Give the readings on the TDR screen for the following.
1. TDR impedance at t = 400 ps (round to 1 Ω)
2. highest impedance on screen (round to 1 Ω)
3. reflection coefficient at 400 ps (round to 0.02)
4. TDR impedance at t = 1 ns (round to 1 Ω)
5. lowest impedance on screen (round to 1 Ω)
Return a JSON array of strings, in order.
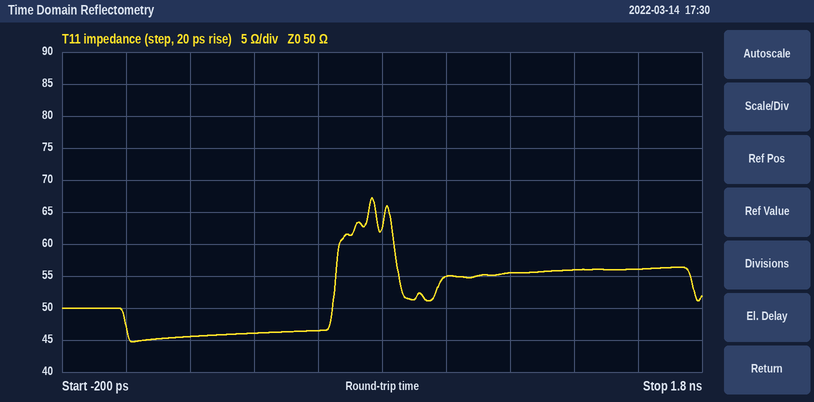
["46 Ω", "67 Ω", "-0.04", "55 Ω", "45 Ω"]
